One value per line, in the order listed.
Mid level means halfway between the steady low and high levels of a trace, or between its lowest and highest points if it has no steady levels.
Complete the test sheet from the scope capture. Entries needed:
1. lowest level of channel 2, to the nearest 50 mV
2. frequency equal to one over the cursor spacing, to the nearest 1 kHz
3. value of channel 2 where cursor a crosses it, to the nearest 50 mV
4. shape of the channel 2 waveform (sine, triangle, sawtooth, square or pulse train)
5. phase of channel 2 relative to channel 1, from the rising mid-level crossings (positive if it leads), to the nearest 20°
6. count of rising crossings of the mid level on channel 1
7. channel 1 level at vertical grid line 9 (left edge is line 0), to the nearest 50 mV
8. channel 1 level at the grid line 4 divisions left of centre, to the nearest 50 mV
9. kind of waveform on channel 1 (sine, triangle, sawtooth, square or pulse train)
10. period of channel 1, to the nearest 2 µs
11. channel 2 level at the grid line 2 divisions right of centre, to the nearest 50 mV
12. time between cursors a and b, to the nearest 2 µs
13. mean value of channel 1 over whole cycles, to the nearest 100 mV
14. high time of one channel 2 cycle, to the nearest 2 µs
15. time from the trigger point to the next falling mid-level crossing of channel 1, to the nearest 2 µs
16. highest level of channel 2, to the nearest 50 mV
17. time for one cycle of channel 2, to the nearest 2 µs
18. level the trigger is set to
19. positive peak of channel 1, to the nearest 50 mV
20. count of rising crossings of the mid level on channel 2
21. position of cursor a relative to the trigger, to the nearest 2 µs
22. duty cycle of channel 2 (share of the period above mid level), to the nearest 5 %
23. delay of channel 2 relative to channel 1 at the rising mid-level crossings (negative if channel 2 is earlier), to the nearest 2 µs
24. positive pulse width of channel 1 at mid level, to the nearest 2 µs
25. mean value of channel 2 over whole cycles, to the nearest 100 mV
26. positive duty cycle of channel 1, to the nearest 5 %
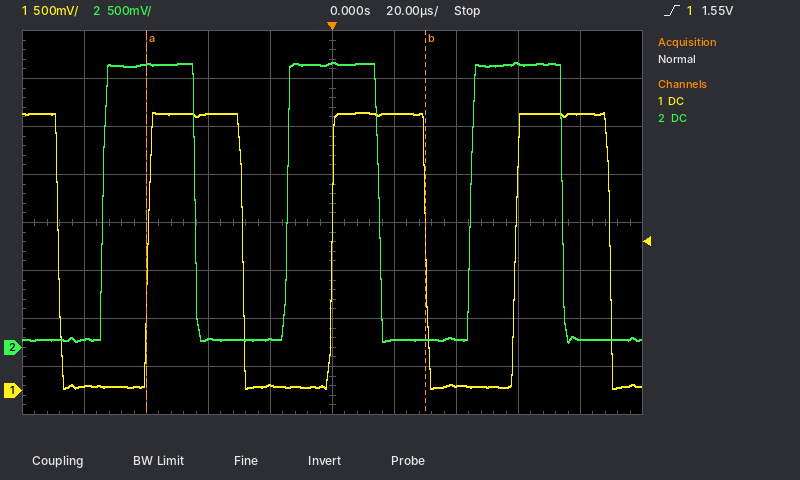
50 mV
11 kHz
2.95 V
square
+80°
3
2.90 V
50 mV
square
60 µs
100 mV
90 µs
1.5 V
30 µs
30 µs
2.95 V
60 µs
1.55 V
2.90 V
3
-60 µs
50 %
-14 µs
30 µs
1.5 V
50 %
